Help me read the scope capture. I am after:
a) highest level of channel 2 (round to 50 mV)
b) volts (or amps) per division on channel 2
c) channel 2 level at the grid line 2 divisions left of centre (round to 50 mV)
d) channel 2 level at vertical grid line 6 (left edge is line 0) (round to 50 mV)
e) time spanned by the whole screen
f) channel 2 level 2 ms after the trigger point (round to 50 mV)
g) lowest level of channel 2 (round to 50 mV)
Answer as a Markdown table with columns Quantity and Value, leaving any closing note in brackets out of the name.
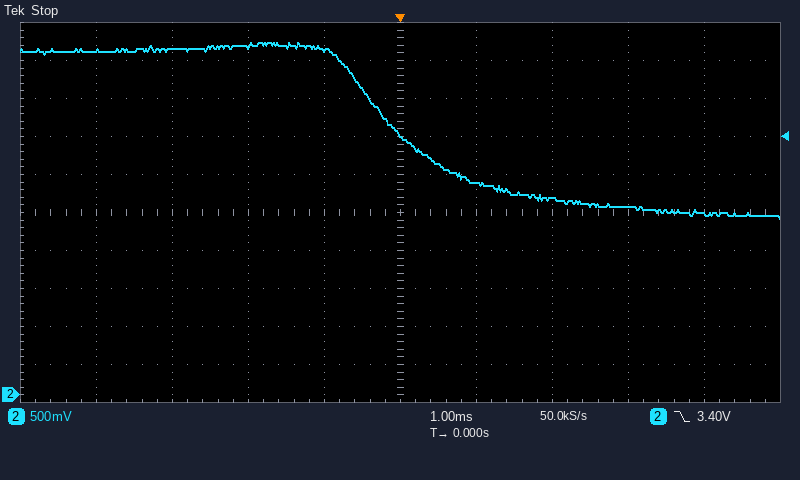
| Quantity | Value |
|---|---|
| highest level of channel 2 | 4.65 V |
| volts (or amps) per division on channel 2 | 500 mV |
| channel 2 level at the grid line 2 divisions left of centre | 4.60 V |
| channel 2 level at vertical grid line 6 (left edge is line 0) | 2.80 V |
| time spanned by the whole screen | 10 ms |
| channel 2 level 2 ms after the trigger point | 2.60 V |
| lowest level of channel 2 | 2.30 V |
